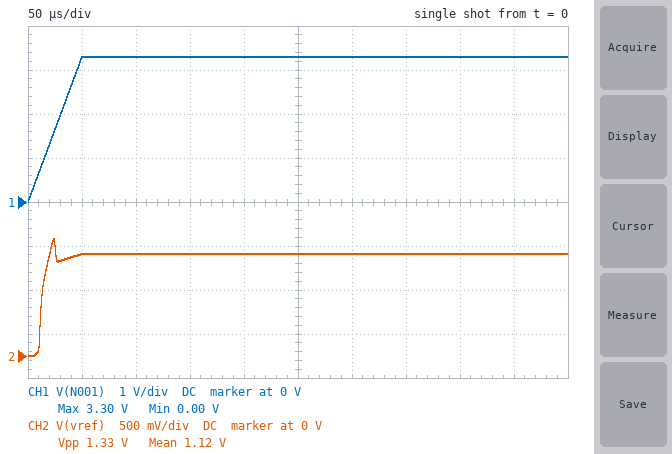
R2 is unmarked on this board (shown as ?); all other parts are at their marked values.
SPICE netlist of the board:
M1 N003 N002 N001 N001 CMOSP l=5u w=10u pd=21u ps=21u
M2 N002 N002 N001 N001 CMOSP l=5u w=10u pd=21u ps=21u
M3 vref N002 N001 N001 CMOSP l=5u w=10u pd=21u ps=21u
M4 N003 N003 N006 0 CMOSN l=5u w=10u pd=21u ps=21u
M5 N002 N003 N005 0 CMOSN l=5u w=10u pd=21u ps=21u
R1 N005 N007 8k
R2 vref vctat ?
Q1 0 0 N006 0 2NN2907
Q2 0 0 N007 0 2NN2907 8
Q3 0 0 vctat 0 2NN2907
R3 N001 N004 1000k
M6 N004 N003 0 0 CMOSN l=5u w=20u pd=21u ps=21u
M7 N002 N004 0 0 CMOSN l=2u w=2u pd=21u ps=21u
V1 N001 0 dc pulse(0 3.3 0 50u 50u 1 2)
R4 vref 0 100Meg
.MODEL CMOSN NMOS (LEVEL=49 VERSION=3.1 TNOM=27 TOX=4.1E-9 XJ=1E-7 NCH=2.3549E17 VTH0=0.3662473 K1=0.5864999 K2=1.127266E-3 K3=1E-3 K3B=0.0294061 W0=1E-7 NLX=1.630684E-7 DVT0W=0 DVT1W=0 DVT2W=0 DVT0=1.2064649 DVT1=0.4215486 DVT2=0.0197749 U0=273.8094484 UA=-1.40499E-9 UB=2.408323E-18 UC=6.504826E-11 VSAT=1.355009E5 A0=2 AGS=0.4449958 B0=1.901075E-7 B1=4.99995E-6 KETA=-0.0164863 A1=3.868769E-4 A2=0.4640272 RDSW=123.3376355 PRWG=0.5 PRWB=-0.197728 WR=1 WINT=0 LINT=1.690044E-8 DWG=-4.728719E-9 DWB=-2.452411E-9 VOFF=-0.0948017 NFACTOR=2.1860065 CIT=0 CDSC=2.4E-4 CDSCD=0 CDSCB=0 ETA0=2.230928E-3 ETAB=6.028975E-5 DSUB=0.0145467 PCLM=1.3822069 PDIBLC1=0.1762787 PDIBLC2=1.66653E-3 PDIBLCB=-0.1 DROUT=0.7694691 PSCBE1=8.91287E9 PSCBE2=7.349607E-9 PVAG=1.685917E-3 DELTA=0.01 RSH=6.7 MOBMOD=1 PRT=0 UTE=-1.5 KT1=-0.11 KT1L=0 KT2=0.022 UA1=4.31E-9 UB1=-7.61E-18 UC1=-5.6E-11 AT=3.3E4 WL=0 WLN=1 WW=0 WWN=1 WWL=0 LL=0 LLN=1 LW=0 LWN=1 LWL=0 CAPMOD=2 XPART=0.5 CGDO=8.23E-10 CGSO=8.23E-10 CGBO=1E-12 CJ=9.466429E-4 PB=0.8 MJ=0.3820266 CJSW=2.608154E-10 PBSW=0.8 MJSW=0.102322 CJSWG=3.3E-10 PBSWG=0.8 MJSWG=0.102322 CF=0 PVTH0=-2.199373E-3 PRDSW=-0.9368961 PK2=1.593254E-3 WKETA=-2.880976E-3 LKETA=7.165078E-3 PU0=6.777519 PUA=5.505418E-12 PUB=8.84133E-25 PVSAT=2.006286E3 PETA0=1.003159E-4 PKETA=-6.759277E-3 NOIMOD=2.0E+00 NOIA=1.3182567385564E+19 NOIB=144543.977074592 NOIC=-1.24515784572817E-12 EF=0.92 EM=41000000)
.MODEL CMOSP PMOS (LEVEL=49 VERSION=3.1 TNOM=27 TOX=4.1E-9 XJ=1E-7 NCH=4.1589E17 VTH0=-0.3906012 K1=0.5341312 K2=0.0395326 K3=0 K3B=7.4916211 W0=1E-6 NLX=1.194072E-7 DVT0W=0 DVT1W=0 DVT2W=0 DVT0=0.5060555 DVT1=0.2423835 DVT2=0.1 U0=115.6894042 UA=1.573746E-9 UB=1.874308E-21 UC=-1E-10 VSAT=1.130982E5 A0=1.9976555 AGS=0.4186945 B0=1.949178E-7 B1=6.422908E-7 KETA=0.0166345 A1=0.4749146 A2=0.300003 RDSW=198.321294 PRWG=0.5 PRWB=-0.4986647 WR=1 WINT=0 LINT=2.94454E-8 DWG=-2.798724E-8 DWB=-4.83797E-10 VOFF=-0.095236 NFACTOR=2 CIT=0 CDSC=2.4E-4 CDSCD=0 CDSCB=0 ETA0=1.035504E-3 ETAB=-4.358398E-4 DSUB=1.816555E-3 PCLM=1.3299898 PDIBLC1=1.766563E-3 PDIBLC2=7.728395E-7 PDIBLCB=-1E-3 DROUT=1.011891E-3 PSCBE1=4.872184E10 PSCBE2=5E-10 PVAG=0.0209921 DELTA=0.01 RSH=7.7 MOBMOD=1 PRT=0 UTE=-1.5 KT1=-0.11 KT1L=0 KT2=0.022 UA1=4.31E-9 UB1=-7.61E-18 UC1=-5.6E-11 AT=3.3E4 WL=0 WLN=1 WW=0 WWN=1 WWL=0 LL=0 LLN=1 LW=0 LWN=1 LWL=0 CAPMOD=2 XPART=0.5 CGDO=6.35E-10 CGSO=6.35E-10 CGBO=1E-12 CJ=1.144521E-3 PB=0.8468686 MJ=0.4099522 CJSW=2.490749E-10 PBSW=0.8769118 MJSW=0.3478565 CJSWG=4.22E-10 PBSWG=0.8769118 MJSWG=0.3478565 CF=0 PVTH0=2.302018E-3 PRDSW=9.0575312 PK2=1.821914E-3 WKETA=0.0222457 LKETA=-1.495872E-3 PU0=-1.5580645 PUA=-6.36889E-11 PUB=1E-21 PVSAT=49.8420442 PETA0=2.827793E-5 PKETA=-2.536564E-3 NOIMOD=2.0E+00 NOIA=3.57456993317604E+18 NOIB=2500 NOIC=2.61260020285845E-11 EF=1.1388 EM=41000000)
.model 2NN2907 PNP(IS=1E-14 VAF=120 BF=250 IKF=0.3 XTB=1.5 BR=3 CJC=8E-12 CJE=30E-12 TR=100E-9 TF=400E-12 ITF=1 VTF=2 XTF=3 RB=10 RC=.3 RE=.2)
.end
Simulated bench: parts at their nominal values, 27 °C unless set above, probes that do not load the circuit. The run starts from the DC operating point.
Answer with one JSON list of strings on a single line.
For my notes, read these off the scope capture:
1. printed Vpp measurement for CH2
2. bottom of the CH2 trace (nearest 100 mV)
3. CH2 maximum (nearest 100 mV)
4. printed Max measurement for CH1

["1.33 V", "0 V", "1.3 V", "3.30 V"]
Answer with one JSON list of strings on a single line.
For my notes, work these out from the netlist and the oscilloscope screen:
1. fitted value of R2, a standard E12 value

["82 kΩ"]
